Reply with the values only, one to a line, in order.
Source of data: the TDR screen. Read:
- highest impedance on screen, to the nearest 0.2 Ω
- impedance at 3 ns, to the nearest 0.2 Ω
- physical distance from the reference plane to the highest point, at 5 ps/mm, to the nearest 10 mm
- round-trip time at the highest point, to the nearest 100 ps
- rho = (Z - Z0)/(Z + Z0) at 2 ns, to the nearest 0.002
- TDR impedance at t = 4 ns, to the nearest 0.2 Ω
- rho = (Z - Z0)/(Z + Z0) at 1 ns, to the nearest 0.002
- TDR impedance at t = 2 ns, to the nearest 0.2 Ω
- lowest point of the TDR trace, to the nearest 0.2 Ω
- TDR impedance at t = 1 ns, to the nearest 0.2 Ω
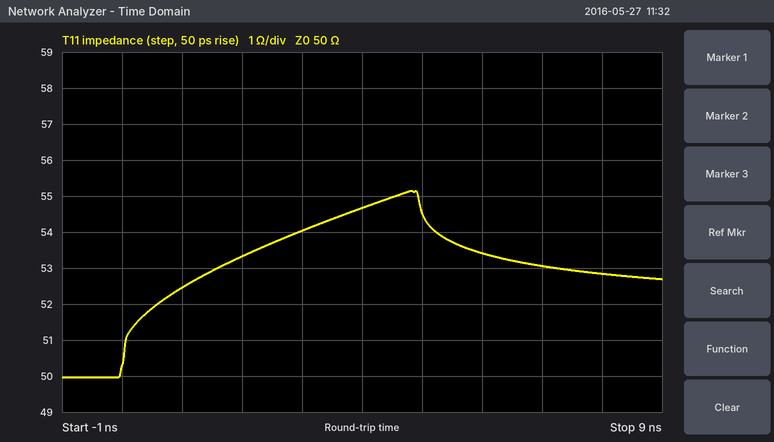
55.2 Ω
54.0 Ω
480 mm
4.8 ns
+0.032
54.6 Ω
+0.024
53.4 Ω
50.0 Ω
52.4 Ω
